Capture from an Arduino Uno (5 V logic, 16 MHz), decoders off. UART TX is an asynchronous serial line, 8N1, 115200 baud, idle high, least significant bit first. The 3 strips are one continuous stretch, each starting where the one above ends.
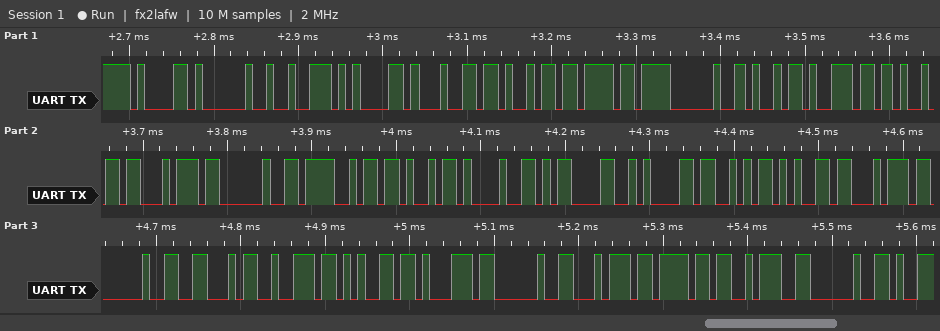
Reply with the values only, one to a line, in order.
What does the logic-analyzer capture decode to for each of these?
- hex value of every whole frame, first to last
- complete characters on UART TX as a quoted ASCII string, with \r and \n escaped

61 20 72 61 64 69 6F 20 69 6E 69 74 20 4F 4B 21 0D 0A 53 65 74 20 46 72 65 71 20 74 6F 3A 20
"a radio init OK!\r\nSet Freq to: "
